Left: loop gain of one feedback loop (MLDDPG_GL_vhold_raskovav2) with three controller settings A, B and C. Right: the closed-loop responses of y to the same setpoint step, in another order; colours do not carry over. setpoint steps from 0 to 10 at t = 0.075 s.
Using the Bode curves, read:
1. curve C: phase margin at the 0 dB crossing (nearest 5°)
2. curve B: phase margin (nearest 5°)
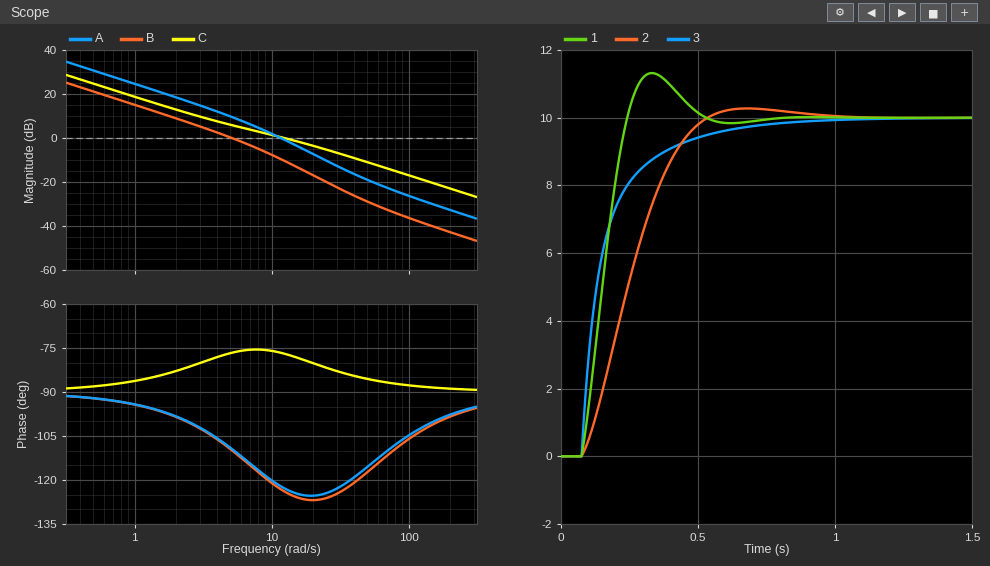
105°
70°
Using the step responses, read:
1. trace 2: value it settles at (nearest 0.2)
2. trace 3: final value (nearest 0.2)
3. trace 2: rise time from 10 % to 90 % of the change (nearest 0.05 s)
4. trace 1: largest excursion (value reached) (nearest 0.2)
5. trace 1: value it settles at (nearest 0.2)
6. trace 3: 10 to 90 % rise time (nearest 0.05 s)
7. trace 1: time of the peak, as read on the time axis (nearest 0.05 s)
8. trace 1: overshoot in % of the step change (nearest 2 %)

10.0
10.0
0.30 s
11.4
10.0
0.30 s
0.35 s
14 %
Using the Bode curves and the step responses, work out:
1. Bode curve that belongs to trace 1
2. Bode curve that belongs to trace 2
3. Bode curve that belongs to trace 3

A
B
C
